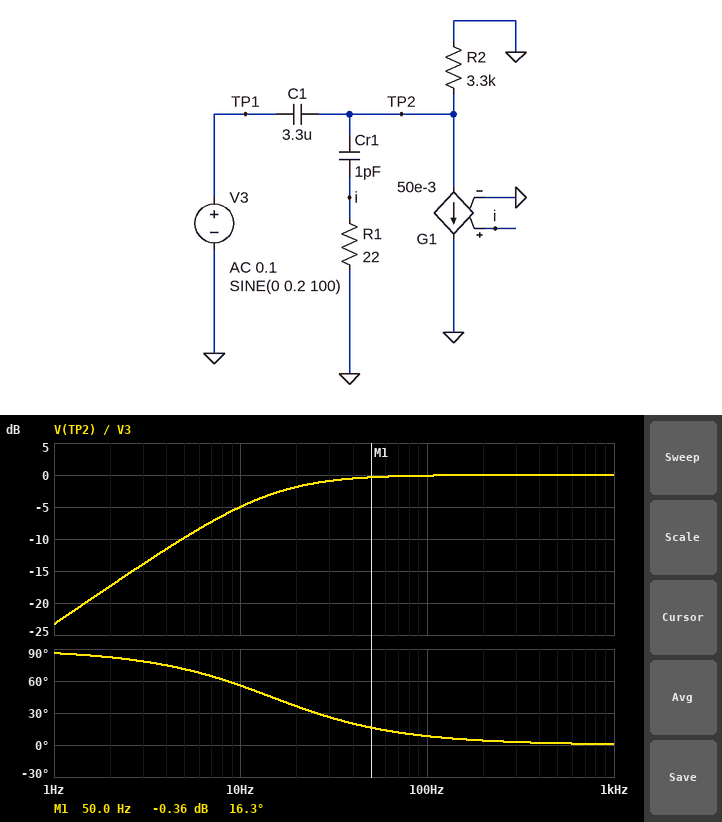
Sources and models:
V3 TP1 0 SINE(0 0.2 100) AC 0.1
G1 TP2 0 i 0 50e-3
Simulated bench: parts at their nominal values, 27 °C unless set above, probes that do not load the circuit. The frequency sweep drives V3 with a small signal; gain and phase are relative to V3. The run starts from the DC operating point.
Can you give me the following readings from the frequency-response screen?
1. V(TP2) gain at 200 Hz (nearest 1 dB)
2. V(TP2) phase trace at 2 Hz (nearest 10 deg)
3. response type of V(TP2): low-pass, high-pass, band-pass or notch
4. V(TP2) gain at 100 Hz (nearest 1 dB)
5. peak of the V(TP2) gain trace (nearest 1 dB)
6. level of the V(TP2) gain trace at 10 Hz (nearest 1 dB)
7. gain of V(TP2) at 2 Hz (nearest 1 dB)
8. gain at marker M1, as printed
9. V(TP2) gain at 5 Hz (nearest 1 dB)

0 dB
80 deg
high-pass
0 dB
0 dB
-5 dB
-17 dB
-0.36 dB
-10 dB
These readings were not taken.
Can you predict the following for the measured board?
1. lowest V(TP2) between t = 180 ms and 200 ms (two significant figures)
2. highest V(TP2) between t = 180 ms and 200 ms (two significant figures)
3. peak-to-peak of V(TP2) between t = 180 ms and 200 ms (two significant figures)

-200 mV
200 mV
400 mV
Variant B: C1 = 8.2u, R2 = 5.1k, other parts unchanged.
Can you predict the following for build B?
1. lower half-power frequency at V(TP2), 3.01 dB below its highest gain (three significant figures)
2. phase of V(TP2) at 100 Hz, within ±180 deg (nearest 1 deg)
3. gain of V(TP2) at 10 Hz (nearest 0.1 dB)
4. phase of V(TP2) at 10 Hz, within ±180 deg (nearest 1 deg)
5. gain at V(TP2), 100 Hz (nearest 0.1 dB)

3.81 Hz
2 deg
-0.6 dB
21 deg
0 dB
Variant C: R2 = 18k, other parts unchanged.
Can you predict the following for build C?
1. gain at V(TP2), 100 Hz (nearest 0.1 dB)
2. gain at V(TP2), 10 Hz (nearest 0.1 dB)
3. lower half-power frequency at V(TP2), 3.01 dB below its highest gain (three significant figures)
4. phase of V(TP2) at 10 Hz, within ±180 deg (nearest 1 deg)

0 dB
-0.3 dB
2.68 Hz
15 deg
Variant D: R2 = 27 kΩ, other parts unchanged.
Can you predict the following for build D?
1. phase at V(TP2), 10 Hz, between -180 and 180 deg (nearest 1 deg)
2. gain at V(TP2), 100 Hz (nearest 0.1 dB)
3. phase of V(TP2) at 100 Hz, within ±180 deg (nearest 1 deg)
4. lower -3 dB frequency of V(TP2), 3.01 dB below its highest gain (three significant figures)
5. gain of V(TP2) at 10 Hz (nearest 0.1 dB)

10 deg
0 dB
1 deg
1.79 Hz
-0.1 dB
